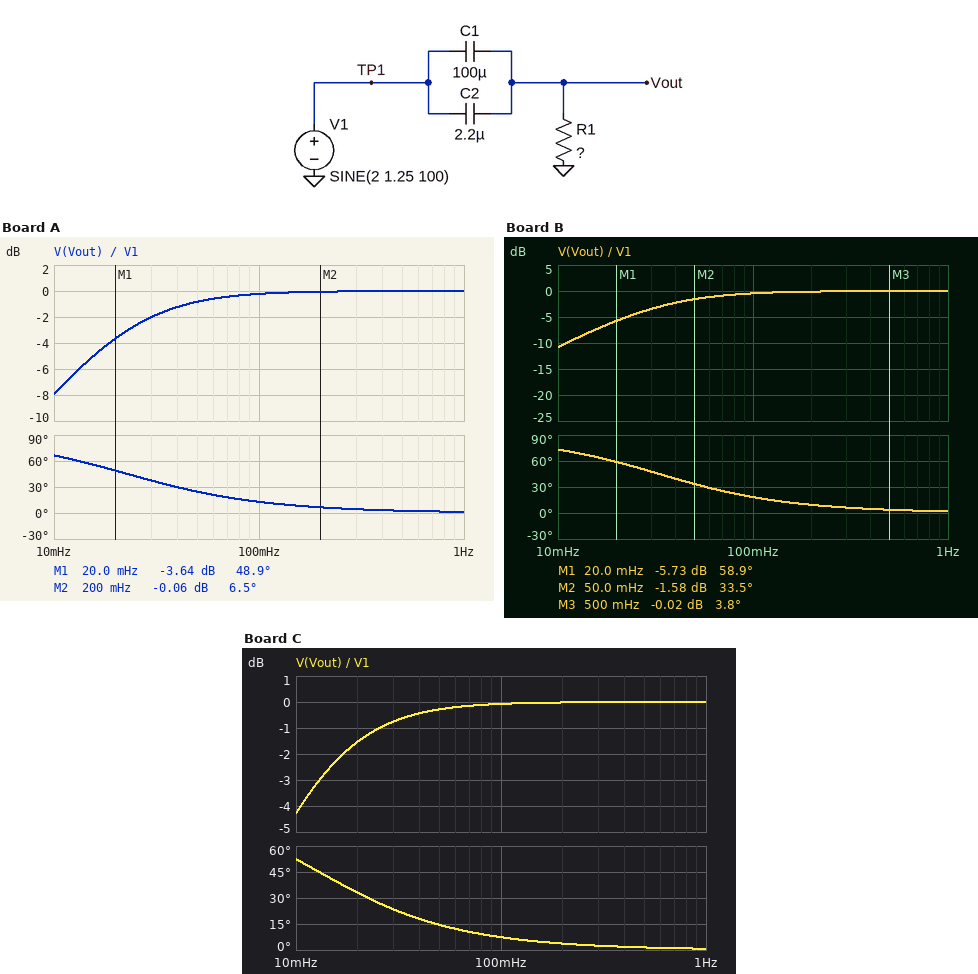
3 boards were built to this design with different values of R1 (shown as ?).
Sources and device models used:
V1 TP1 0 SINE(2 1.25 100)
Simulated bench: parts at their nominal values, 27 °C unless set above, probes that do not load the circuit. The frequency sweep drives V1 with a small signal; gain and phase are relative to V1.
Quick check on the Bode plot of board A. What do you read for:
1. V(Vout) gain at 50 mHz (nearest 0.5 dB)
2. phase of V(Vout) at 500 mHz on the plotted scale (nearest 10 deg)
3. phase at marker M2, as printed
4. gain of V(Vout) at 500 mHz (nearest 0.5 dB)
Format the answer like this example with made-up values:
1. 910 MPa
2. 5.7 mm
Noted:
1. -1.0 dB
2. 0 deg
3. 6.5 deg
4. 0 dB
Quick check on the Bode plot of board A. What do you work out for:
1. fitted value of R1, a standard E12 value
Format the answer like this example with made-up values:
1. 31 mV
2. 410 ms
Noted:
1. 68 kΩ
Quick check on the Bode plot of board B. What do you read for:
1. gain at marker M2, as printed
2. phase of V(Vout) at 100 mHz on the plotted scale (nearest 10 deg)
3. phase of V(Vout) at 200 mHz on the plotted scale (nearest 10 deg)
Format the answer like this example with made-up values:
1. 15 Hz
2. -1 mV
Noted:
1. -1.58 dB
2. 20 deg
3. 10 deg
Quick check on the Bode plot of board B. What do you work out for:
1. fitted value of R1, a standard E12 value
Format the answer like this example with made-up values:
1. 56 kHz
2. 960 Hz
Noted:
1. 47 kΩ
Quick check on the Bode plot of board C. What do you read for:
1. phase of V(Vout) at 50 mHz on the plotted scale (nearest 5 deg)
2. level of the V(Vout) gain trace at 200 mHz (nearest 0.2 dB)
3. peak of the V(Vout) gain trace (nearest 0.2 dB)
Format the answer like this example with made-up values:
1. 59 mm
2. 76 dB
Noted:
1. 15 deg
2. 0 dB
3. 0 dB
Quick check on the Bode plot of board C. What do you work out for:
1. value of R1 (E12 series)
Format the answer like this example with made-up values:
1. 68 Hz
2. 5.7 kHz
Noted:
1. 120 kΩ
